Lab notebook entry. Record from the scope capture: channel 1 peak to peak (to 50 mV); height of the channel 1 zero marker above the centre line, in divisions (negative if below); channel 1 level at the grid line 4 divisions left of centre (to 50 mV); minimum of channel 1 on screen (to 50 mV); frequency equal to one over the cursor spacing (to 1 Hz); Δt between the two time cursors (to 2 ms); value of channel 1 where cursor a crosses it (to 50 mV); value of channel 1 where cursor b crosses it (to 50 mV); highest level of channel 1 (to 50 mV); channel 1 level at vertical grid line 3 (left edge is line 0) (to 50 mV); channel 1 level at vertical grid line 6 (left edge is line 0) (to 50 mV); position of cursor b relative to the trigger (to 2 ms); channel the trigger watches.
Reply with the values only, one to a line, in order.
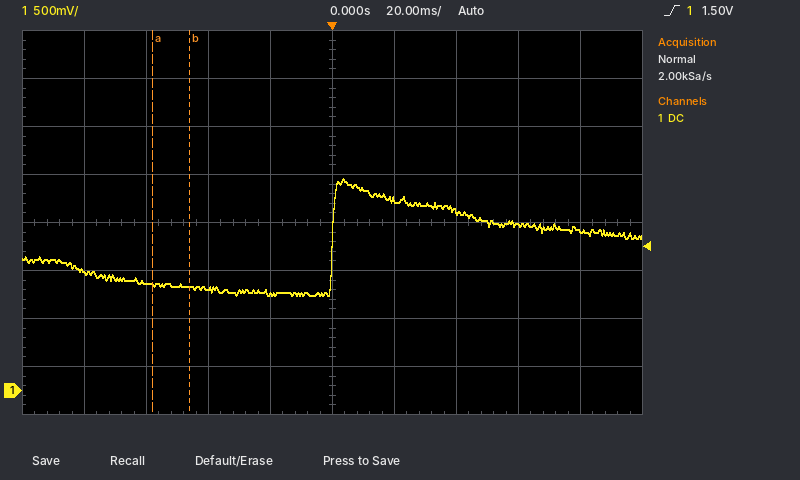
1.20 V
-3.5 div
1.25 V
1.00 V
83 Hz
12 ms
1.10 V
1.10 V
2.20 V
1.05 V
2.00 V
-46 ms
channel 1
